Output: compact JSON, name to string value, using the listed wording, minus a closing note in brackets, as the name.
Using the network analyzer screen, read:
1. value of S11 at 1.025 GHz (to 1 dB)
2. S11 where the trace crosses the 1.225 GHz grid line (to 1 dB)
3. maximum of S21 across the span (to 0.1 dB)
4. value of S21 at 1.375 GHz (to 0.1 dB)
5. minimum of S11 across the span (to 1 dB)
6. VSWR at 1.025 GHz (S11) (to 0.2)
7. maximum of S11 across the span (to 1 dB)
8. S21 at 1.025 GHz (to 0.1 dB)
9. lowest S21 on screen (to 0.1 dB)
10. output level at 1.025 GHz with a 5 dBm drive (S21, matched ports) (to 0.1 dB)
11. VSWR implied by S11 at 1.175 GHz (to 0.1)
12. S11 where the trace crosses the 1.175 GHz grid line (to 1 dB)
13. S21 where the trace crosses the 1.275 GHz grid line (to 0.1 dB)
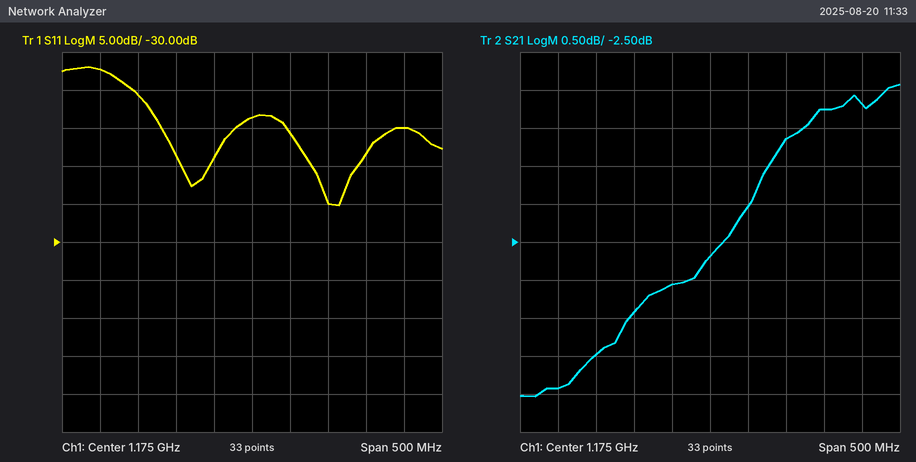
{"value of S11 at 1.025 GHz": "-11 dB", "S11 where the trace crosses the 1.225 GHz grid line": "-16 dB", "maximum of S21 across the span": "-0.4 dB", "value of S21 at 1.375 GHz": "-0.7 dB", "minimum of S11 across the span": "-25 dB", "VSWR at 1.025 GHz (S11)": "1.8", "maximum of S11 across the span": "-7 dB", "S21 at 1.025 GHz": "-4.0 dB", "lowest S21 on screen": "-4.5 dB", "output level at 1.025 GHz with a 5 dBm drive (S21, matched ports)": "1.0 dBm", "VSWR implied by S11 at 1.175 GHz": "1.5", "S11 where the trace crosses the 1.175 GHz grid line": "-14 dB", "S21 where the trace crosses the 1.275 GHz grid line": "-1.1 dB"}
